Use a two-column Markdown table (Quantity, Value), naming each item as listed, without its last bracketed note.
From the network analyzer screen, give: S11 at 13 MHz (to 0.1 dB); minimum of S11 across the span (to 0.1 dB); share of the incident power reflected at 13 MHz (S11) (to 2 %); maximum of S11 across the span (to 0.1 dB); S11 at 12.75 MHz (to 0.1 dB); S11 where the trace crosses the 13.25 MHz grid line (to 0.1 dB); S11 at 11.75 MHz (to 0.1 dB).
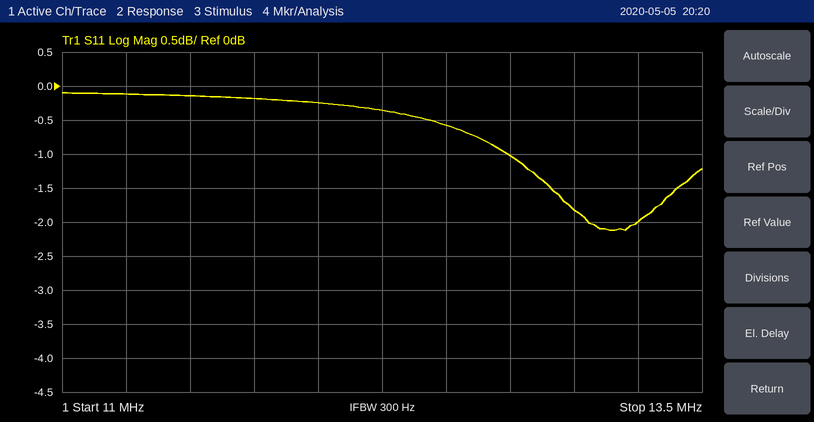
| Quantity | Value |
|---|---|
| S11 at 13 MHz | -1.8 dB |
| minimum of S11 across the span | -2.1 dB |
| share of the incident power reflected at 13 MHz (S11) | 66 % |
| maximum of S11 across the span | -0.1 dB |
| S11 at 12.75 MHz | -1.0 dB |
| S11 where the trace crosses the 13.25 MHz grid line | -2.0 dB |
| S11 at 11.75 MHz | -0.2 dB |
